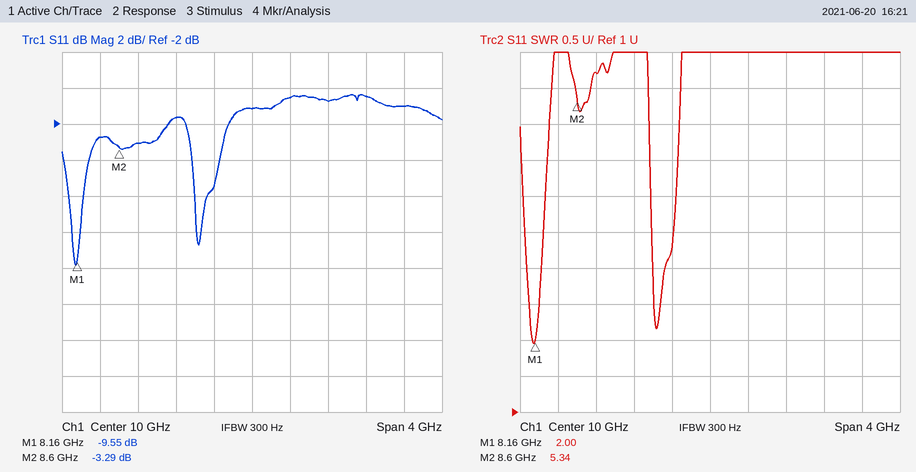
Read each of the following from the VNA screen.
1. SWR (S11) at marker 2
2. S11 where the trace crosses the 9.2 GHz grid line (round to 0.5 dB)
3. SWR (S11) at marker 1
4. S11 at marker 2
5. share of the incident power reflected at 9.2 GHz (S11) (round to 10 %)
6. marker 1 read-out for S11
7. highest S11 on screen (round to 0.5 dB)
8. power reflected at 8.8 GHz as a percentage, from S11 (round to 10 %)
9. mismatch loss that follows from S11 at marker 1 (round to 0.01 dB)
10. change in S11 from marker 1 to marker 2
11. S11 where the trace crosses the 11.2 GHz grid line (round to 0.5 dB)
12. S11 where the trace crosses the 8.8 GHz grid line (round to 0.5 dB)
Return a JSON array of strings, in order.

["5.34", "-1.5 dB", "2.00", "-3.29 dB", "70 %", "-9.55 dB", "-0.5 dB", "50 %", "0.51 dB", "6.26 dB", "-0.5 dB", "-3.0 dB"]
